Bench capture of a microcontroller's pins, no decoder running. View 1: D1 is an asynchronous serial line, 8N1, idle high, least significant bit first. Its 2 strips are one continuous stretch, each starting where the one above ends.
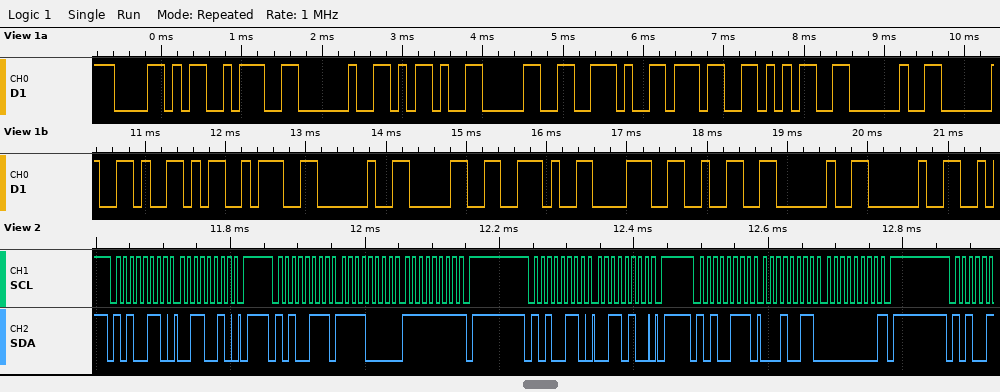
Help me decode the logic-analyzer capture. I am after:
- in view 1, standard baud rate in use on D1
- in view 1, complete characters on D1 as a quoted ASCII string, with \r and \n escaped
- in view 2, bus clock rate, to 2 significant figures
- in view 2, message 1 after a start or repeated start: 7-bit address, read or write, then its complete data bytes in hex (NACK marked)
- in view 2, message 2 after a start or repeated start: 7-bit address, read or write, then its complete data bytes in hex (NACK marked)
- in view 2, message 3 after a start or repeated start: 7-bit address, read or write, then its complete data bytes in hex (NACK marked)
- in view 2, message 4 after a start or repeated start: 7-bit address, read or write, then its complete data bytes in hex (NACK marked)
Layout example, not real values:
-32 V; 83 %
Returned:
9600 baud; "X: -0.75  Y: 0.82  "; 100 kHz; 0x53 write: 32; 0x53 read: F0 FF NACK; 0x53 write: 34; 0x53 read: 13 00 NACK
